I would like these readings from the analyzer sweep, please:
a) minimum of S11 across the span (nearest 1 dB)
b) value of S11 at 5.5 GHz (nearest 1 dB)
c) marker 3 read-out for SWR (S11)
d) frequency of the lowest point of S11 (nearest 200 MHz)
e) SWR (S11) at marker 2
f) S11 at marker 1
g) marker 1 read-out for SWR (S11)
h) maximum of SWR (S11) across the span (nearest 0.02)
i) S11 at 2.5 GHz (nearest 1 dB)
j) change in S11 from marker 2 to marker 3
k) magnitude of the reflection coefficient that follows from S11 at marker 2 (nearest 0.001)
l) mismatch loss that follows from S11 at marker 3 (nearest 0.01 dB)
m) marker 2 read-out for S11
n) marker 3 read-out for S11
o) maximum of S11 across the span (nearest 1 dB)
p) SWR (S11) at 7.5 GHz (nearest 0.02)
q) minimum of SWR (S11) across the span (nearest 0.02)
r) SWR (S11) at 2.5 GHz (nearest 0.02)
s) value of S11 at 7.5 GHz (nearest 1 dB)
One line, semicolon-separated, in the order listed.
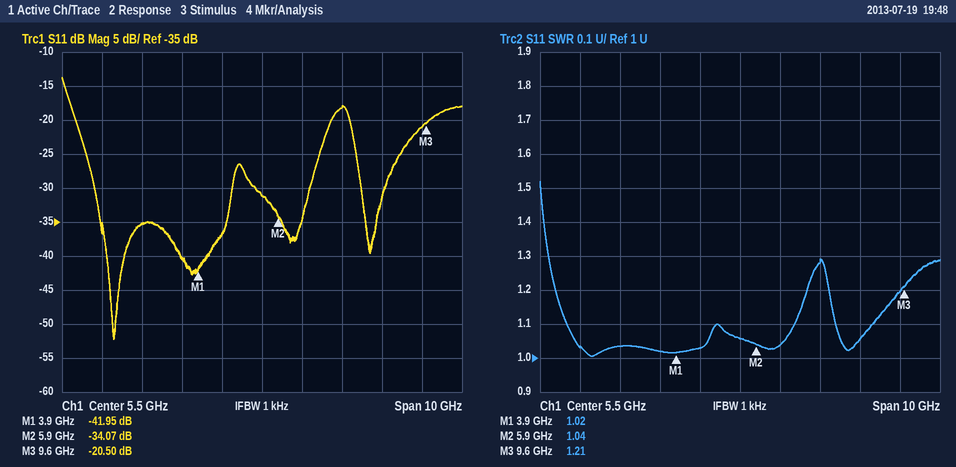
-52 dB; -31 dB; 1.21; 1.8 GHz; 1.04; -41.95 dB; 1.02; 1.52; -35 dB; 13.57 dB; 0.020; 0.04 dB; -34.07 dB; -20.50 dB; -14 dB; 1.28; 1.00; 1.04; -18 dB
